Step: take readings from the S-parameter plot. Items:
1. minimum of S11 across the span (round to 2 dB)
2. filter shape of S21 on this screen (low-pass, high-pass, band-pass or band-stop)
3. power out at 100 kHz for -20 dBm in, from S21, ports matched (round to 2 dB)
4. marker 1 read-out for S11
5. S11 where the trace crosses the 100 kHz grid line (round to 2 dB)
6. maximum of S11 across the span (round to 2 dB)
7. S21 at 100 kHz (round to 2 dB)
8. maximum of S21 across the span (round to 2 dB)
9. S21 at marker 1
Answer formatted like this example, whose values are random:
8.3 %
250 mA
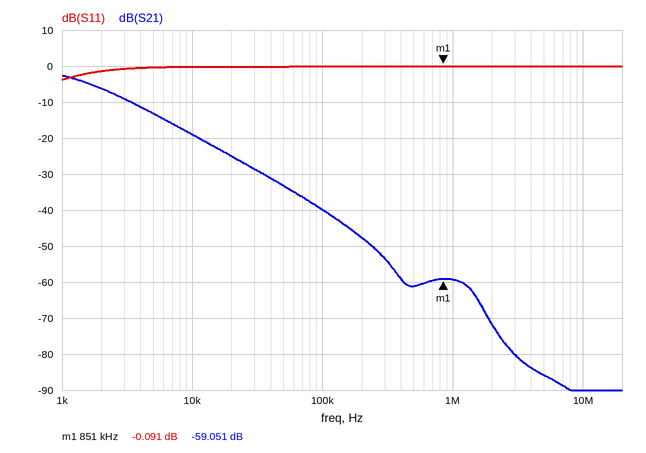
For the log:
-4 dB
low-pass
-60 dBm
-0.091 dB
0 dB
0 dB
-40 dB
-2 dB
-59.051 dB
